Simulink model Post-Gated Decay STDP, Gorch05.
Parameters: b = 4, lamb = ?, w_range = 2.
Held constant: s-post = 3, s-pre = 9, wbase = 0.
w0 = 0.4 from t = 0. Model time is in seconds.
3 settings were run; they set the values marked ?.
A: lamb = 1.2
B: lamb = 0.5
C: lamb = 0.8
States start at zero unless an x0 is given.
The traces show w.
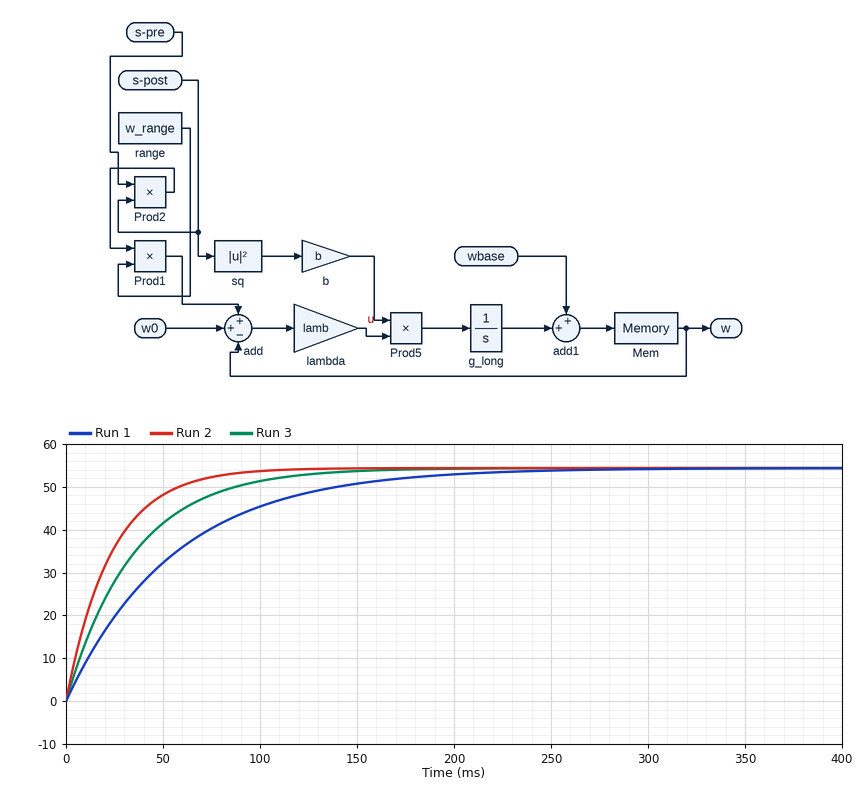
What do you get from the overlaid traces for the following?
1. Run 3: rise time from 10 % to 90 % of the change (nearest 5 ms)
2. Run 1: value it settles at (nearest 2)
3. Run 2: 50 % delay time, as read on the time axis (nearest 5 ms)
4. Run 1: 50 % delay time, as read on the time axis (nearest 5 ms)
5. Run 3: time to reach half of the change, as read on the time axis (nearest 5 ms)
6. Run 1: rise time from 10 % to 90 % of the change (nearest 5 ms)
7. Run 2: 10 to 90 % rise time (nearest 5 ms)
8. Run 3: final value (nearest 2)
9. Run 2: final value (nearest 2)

75 ms
54
15 ms
40 ms
25 ms
120 ms
50 ms
54
54
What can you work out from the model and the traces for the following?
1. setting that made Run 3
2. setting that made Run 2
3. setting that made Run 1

C
A
B
